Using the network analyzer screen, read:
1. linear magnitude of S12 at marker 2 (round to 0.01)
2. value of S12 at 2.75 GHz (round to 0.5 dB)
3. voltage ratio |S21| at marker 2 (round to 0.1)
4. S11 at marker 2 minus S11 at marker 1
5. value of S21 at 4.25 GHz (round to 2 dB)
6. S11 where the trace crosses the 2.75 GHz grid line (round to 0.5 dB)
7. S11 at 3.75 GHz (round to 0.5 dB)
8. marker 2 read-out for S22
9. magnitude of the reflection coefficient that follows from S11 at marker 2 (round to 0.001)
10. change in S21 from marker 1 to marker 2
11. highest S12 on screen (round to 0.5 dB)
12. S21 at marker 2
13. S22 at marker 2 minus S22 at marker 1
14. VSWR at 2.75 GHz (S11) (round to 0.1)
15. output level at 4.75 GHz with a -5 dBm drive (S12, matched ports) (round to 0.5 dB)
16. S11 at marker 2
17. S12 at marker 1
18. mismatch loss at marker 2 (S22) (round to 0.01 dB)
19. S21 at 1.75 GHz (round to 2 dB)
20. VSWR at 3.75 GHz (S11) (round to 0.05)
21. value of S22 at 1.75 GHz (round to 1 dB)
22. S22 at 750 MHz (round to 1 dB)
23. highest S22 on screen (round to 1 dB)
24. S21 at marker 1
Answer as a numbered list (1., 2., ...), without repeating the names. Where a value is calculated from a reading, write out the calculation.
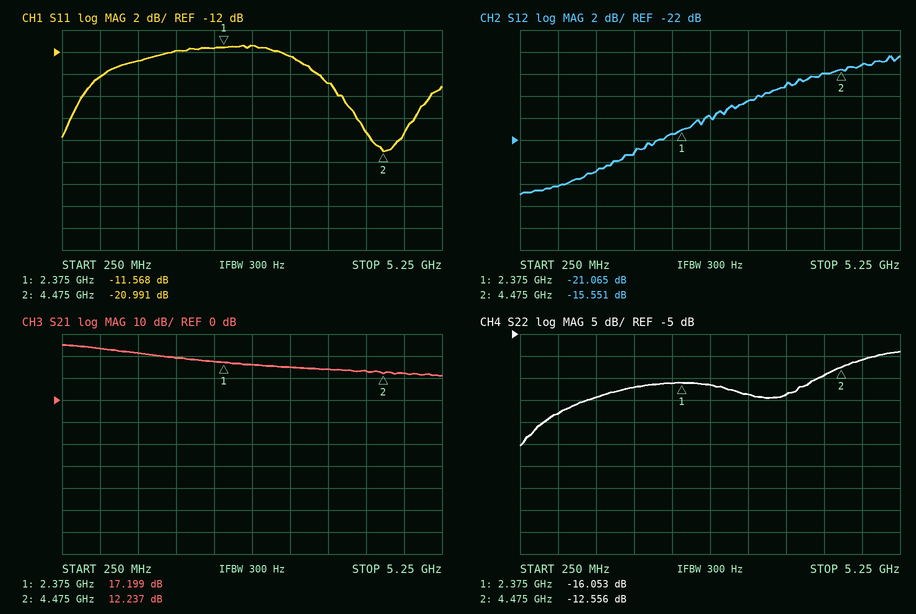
1. 10^(-15.551/20) ≈ 0.17
2. -20.0 dB
3. 10^(12.237/20) ≈ 4.1
4. -20.991 − (-11.568) = -9.423 dB
5. 14 dB
6. -11.5 dB
7. -15.0 dB
8. -12.556 dB
9. 10^(-20.991/20) ≈ 0.089
10. 12.237 − (17.199) = -4.962 dB
11. -14.5 dB
12. 12.237 dB
13. -12.556 − (-16.053) = 3.497 dB
14. |Γ| = 10^(-11.5/20) = 0.2661; VSWR = (1 + 0.2661)/(1 − 0.2661) ≈ 1.7
15. -5 dBm + (-15.0 dB) = -20.0 dBm
16. -20.991 dB
17. -21.065 dB
18. −10 log10(1 − 10^(-12.556/10)) ≈ 0.25 dB
19. 20 dB
20. |Γ| = 10^(-15/20) = 0.1778; VSWR = (1 + 0.1778)/(1 − 0.1778) ≈ 1.43, so 1.45 to the nearest 0.05
21. -17 dB
22. -23 dB
23. -9 dB
24. 17.199 dB
